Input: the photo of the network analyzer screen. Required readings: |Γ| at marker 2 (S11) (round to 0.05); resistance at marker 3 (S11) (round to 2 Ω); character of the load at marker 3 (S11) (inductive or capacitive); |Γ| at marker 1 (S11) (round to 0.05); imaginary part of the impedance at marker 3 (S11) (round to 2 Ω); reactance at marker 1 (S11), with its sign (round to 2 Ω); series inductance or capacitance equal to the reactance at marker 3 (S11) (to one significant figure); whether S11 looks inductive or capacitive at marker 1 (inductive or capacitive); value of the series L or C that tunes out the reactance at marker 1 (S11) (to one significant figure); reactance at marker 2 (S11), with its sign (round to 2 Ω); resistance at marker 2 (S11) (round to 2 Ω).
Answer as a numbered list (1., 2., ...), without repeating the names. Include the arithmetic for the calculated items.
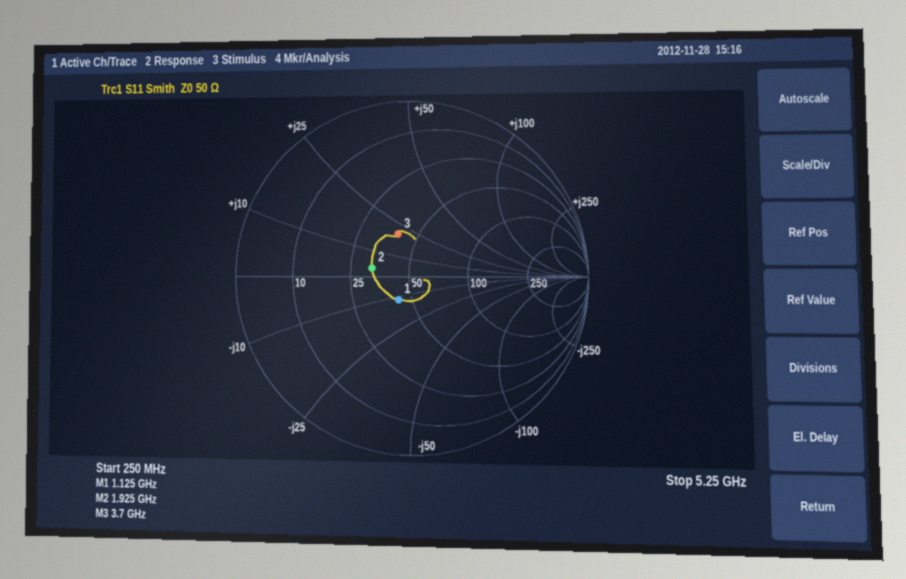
1. 0.20
2. 40 Ω
3. inductive
4. 0.15
5. +20 Ω
6. -12 Ω
7. L = 20 Ω/(2π × 3.7 GHz) ≈ 860 pH, so 900 pH to one significant figure
8. capacitive
9. L = 12 Ω/(2π × 1.125 GHz) ≈ 2 nH
10. +4 Ω
11. 32 Ω
